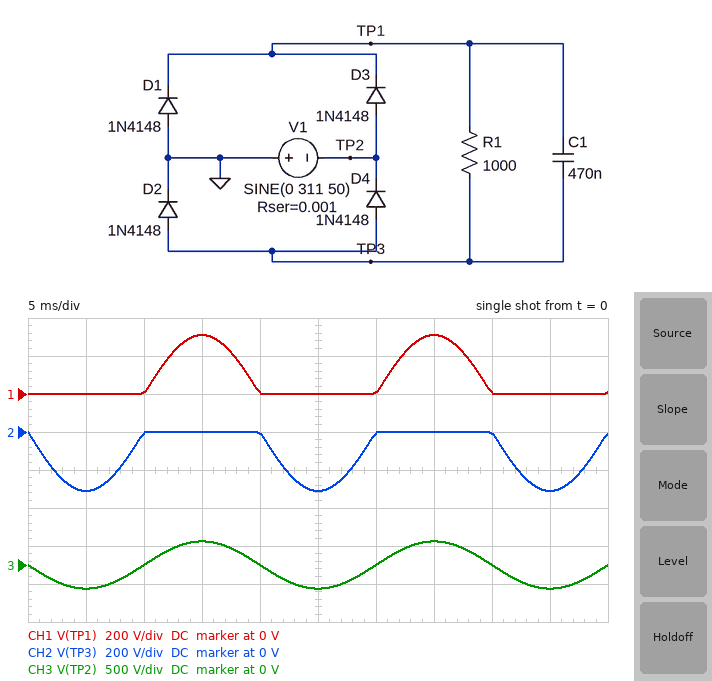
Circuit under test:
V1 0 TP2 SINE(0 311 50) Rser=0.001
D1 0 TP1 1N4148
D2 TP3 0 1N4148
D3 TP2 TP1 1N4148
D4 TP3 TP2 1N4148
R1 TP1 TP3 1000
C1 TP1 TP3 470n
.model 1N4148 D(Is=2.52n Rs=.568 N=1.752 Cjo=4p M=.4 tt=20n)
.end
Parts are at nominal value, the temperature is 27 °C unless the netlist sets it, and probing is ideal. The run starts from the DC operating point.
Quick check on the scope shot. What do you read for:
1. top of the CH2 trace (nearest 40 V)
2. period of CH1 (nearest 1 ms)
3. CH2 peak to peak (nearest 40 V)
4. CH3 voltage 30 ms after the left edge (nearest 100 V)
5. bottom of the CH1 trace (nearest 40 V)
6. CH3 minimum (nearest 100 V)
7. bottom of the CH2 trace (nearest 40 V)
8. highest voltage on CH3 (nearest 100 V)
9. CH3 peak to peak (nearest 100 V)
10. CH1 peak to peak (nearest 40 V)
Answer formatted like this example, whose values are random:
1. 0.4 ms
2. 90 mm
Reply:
1. 0 V
2. 20 ms
3. 320 V
4. 0 V
5. 0 V
6. -300 V
7. -320 V
8. 300 V
9. 600 V
10. 320 V
